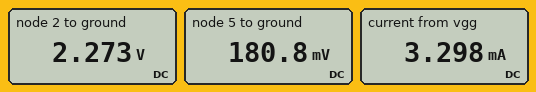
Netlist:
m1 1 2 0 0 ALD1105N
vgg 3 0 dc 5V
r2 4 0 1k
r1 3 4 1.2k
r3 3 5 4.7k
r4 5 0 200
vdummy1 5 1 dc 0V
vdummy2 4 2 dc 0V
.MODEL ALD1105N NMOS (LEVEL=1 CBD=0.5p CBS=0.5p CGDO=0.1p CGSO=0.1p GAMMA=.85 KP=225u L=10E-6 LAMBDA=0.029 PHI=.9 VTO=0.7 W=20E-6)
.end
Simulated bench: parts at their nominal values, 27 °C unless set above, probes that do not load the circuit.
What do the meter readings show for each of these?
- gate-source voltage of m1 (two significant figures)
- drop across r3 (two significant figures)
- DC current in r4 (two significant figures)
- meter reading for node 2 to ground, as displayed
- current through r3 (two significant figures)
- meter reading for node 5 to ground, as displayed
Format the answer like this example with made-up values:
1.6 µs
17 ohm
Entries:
2.3 V
4.8 V
900 µA
2.273 V
1.0 mA
180.8 mV
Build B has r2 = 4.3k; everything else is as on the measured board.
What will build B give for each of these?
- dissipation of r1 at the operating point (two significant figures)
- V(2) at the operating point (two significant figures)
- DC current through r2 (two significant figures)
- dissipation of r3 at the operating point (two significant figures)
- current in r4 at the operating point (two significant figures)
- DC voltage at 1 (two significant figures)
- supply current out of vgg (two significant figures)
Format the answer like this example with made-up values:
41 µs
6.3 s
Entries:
990 µW
3.9 V
910 µA
5.0 mW
800 µA
160 mV
1.9 mA
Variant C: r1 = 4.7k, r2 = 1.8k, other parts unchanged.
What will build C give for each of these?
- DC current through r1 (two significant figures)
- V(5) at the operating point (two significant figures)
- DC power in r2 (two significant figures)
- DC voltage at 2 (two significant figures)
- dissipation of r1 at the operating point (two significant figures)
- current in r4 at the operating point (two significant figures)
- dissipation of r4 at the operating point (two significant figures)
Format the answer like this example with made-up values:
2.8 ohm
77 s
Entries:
770 µA
190 mV
1.1 mW
1.4 V
2.8 mW
970 µA
190 µW
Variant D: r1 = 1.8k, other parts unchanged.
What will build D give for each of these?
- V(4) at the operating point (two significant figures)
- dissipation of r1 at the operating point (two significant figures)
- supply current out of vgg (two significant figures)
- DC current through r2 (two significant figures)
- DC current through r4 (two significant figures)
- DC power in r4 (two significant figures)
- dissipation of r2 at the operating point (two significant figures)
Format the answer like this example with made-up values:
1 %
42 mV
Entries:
1.8 V
5.7 mW
2.8 mA
1.8 mA
940 µA
180 µW
3.2 mW
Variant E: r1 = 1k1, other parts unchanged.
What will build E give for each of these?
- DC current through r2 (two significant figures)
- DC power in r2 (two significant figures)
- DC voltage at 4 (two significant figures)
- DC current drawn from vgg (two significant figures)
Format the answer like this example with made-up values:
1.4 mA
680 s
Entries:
2.4 mA
5.7 mW
2.4 V
3.4 mA
